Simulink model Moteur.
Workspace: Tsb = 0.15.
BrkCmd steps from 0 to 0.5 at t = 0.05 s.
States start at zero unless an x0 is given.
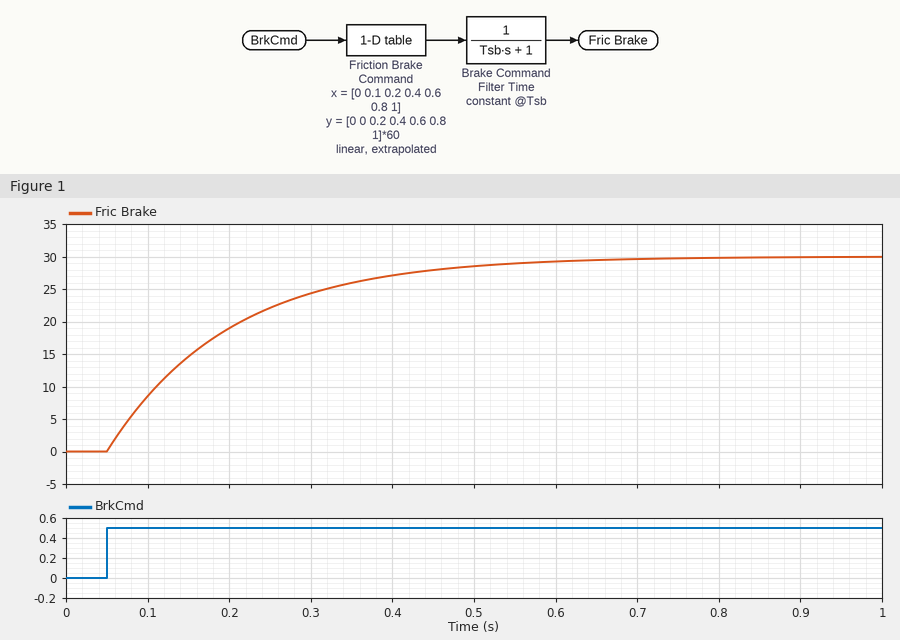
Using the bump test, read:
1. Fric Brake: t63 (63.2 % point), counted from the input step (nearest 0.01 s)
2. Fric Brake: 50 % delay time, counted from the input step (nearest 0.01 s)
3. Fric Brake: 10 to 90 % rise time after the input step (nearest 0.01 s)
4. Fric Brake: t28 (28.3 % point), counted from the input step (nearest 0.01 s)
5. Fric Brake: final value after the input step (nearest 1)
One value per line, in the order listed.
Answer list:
0.15 s
0.10 s
0.33 s
0.05 s
30
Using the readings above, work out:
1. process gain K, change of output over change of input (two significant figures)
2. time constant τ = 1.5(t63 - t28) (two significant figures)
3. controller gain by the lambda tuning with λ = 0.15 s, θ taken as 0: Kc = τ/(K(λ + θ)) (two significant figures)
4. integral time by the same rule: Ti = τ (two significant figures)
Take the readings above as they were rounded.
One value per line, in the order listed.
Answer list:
60
0.15 s
0.017
0.15 s
